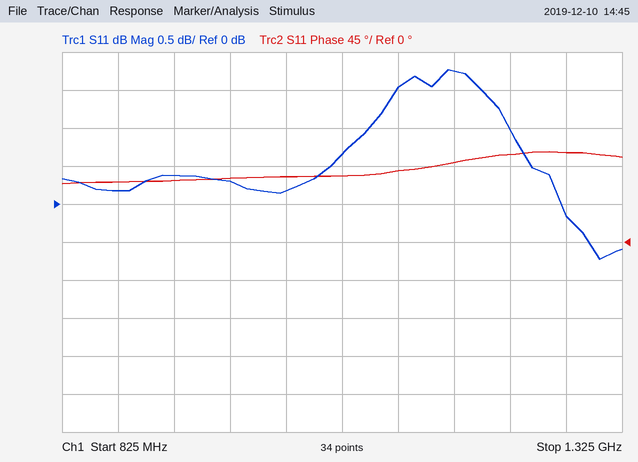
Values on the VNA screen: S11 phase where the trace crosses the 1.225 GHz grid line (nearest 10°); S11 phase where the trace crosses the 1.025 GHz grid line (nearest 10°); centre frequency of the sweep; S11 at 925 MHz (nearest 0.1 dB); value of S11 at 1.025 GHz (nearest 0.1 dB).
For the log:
100°
80°
1.075 GHz
0.4 dB
0.2 dB
